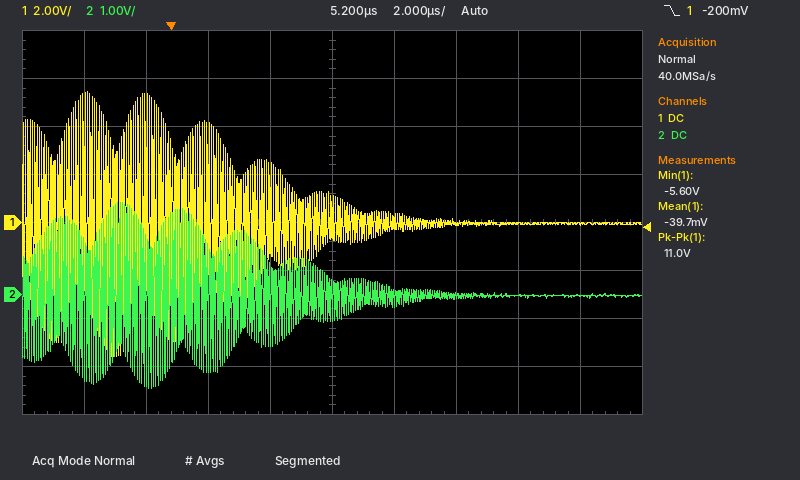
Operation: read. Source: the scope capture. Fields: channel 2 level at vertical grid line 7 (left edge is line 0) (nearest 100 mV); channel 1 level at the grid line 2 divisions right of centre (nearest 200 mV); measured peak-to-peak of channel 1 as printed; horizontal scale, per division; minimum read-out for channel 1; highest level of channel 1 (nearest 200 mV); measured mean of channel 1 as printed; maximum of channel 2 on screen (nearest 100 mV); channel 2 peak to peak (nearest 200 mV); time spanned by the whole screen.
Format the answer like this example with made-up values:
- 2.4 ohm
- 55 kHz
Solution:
- 0.0 V
- 0.0 V
- 11.0 V
- 2 µs
- -5.60 V
- 5.4 V
- -39.7 mV
- 1.9 V
- 3.8 V
- 20 µs
